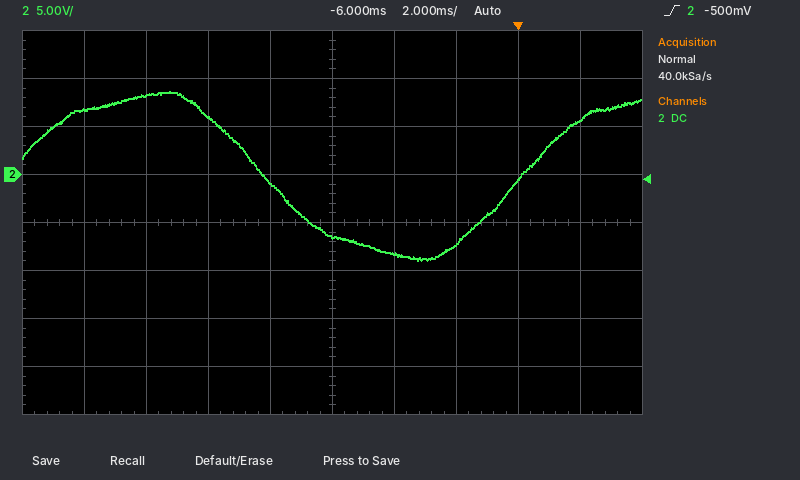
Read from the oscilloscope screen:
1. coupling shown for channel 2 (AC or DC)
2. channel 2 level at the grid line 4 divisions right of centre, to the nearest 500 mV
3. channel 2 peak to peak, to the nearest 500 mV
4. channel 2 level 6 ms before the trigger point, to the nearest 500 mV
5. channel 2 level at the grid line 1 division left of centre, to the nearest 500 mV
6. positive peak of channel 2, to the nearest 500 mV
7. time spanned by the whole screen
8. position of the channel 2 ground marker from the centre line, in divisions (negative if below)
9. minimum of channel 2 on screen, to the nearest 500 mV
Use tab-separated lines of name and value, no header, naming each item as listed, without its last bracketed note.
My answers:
coupling shown for channel 2	DC
channel 2 level at the grid line 4 divisions right of centre, to the nearest 500 mV	5.5 V
channel 2 peak to peak, to the nearest 500 mV	17.5 V
channel 2 level 6 ms before the trigger point, to the nearest 500 mV	-6.5 V
channel 2 level at the grid line 1 division left of centre, to the nearest 500 mV	-1.0 V
positive peak of channel 2, to the nearest 500 mV	8.5 V
time spanned by the whole screen	20 ms
position of the channel 2 ground marker from the centre line, in divisions	+1.0 div
minimum of channel 2 on screen, to the nearest 500 mV	-9.0 V
